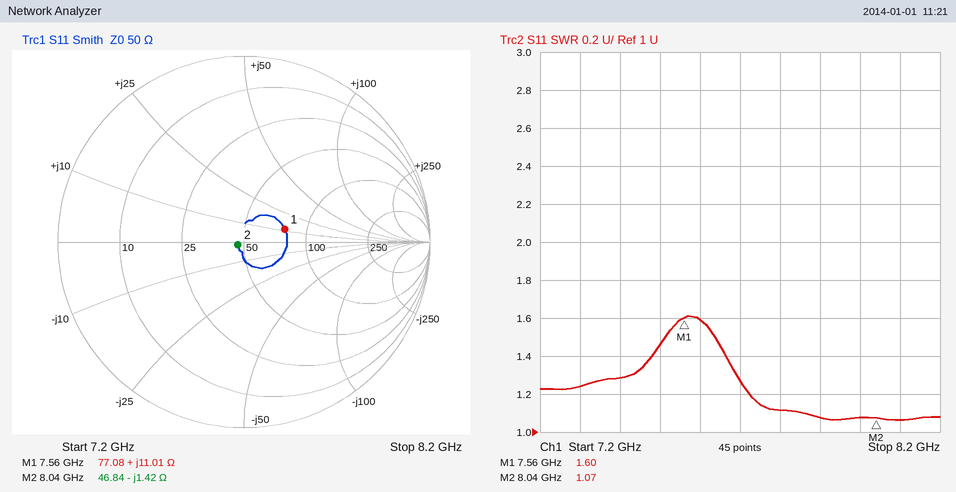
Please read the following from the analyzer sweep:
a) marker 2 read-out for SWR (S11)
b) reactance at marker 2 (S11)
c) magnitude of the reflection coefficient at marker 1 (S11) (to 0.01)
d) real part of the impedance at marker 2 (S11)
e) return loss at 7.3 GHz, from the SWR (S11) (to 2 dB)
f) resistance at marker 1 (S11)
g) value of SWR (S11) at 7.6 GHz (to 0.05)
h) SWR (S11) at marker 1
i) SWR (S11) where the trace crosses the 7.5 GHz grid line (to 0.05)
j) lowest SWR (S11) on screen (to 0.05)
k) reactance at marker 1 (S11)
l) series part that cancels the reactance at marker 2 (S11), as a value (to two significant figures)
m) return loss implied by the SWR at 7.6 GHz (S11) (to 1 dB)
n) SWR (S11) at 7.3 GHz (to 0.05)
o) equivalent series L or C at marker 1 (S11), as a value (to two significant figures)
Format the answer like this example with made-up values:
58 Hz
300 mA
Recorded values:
1.07
-1.42 Ω
0.23
46.84 Ω
20 dB
77.08 Ω
1.60
1.60
1.45
1.05
+11.01 Ω
28 pH
13 dB
1.25
230 pH
